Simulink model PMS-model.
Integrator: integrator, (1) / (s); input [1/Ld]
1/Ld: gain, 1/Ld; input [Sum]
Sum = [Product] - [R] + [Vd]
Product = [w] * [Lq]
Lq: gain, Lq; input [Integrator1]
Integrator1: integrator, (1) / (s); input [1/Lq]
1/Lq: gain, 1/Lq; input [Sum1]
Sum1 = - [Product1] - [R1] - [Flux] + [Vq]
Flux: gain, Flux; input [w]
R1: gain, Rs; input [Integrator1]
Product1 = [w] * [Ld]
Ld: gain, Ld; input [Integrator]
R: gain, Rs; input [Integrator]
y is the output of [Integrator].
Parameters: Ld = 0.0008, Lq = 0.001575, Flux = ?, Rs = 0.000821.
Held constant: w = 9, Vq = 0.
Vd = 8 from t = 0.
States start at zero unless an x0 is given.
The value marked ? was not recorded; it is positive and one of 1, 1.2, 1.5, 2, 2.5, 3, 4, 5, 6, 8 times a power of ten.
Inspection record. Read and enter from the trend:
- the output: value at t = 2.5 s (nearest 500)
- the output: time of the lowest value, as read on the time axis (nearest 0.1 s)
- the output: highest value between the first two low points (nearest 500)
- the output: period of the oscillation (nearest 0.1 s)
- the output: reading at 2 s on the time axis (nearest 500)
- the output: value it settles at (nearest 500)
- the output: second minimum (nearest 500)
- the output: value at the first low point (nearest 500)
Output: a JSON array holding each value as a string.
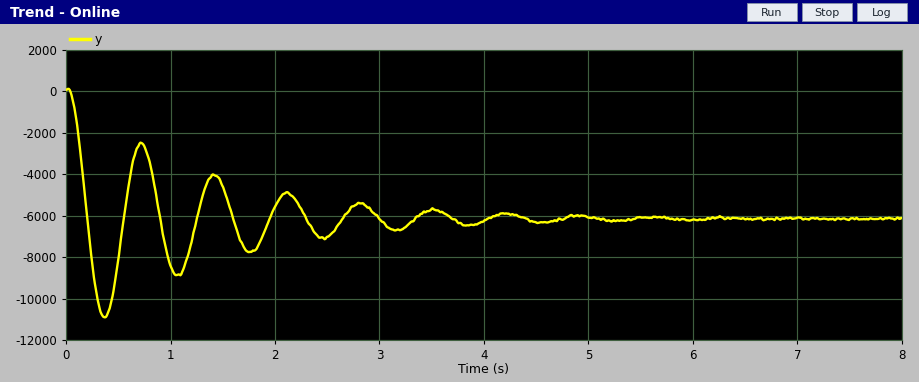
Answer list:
["-7000", "0.4 s", "-2500", "0.7 s", "-5500", "-6000", "-9000", "-11000"]
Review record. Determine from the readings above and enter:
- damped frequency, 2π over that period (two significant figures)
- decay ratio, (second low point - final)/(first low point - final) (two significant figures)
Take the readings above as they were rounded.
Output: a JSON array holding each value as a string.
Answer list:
["9.0 rad/s", "0.60"]
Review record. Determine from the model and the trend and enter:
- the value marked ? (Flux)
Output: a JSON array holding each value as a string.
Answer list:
["5"]
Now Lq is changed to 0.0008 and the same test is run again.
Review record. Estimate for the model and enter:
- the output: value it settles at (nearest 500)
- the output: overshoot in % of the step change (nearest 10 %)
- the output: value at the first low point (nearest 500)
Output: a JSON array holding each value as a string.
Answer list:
["-6000", "70 %", "-10500"]
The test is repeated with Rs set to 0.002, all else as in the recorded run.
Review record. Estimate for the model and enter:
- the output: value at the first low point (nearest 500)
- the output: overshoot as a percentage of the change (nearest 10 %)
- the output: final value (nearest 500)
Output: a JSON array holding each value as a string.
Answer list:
["-9000", "50 %", "-6000"]
